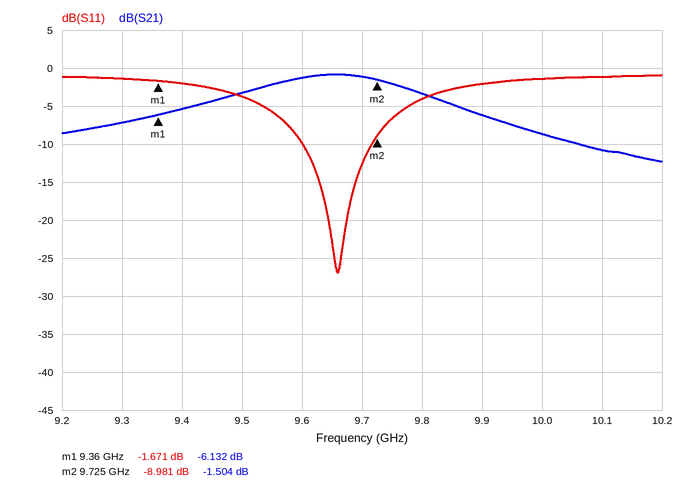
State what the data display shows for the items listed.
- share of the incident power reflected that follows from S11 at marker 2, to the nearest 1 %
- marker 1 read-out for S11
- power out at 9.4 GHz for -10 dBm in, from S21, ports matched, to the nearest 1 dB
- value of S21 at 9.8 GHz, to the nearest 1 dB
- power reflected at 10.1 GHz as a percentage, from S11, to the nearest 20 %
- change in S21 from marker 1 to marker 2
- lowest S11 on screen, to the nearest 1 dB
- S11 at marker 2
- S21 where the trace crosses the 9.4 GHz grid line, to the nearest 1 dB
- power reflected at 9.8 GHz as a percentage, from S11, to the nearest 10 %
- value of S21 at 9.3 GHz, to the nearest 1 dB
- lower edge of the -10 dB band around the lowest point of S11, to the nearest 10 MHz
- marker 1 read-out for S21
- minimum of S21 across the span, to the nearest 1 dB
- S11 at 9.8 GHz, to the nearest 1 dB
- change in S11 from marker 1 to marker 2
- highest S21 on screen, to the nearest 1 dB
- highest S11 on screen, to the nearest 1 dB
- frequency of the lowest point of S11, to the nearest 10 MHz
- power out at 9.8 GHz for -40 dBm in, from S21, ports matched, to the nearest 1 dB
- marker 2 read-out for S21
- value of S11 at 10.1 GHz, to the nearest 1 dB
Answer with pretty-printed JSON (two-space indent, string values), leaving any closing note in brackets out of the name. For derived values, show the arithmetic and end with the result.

{
  "share of the incident power reflected that follows from S11 at marker 2, to the nearest 1 %": "10^(-8.981/10) ≈ 13 %",
  "marker 1 read-out for S11": "-1.671 dB",
  "power out at 9.4 GHz for -10 dBm in, from S21, ports matched, to the nearest 1 dB": "-10 dBm + (-5 dB) = -15 dBm",
  "value of S21 at 9.8 GHz, to the nearest 1 dB": "-3 dB",
  "power reflected at 10.1 GHz as a percentage, from S11, to the nearest 20 %": "10^(-1/10) ≈ 79.4 %, so 80 % to the nearest 20 %",
  "change in S21 from marker 1 to marker 2": "-1.504 − (-6.132) = 4.628 dB",
  "lowest S11 on screen, to the nearest 1 dB": "-27 dB",
  "S11 at marker 2": "-8.981 dB",
  "S21 where the trace crosses the 9.4 GHz grid line, to the nearest 1 dB": "-5 dB",
  "power reflected at 9.8 GHz as a percentage, from S11, to the nearest 10 %": "10^(-4/10) ≈ 40 %",
  "value of S21 at 9.3 GHz, to the nearest 1 dB": "-7 dB",
  "lower edge of the -10 dB band around the lowest point of S11, to the nearest 10 MHz": "9.60 GHz",
  "marker 1 read-out for S21": "-6.132 dB",
  "minimum of S21 across the span, to the nearest 1 dB": "-12 dB",
  "S11 at 9.8 GHz, to the nearest 1 dB": "-4 dB",
  "change in S11 from marker 1 to marker 2": "-8.981 − (-1.671) = -7.310 dB",
  "highest S21 on screen, to the nearest 1 dB": "-1 dB",
  "highest S11 on screen, to the nearest 1 dB": "-1 dB",
  "frequency of the lowest point of S11, to the nearest 10 MHz": "9.66 GHz",
  "power out at 9.8 GHz for -40 dBm in, from S21, ports matched, to the nearest 1 dB": "-40 dBm + (-3 dB) = -43 dBm",
  "marker 2 read-out for S21": "-1.504 dB",
  "value of S11 at 10.1 GHz, to the nearest 1 dB": "-1 dB"
}
